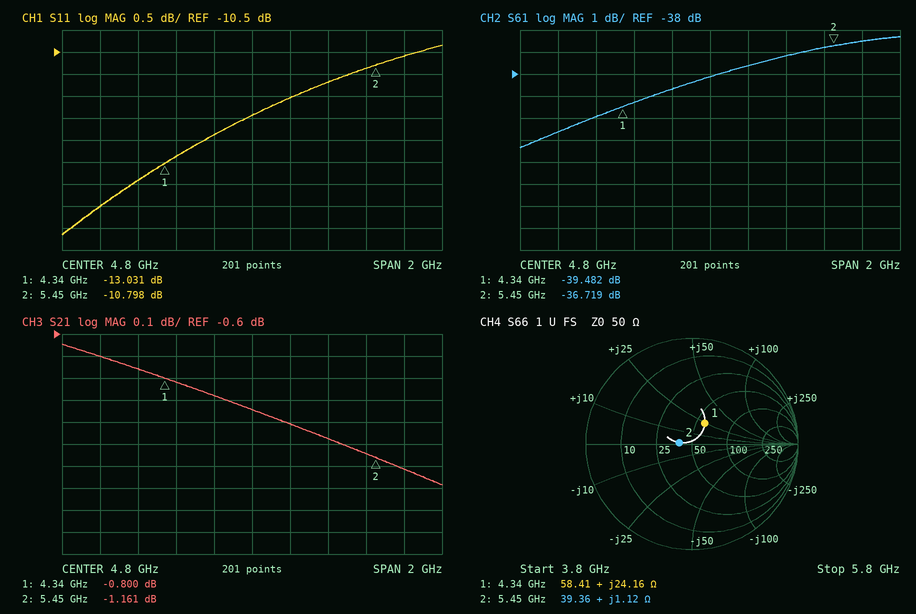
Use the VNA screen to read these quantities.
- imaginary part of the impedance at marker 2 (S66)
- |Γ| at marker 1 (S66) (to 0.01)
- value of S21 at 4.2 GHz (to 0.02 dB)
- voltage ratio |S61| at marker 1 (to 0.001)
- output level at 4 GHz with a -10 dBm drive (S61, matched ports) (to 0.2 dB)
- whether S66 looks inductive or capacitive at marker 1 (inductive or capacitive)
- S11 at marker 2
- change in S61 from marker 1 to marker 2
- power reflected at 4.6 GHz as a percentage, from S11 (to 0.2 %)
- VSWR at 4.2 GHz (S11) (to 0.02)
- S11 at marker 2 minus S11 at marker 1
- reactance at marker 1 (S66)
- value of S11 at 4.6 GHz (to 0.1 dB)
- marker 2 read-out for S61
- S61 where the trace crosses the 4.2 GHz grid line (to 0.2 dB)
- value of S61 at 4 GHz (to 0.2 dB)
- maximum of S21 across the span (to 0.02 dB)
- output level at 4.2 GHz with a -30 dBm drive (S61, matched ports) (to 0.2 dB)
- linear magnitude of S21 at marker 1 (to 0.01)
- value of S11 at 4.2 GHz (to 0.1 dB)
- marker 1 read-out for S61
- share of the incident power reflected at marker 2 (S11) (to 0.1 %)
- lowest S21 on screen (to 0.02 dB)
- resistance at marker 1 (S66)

+1.12 Ω
0.23
-0.76 dB
0.011
-50.6 dBm
inductive
-10.798 dB
2.763 dB
5.8 %
1.54
2.233 dB
+24.16 Ω
-12.4 dB
-36.719 dB
-40.0 dB
-40.6 dB
-0.64 dB
-70.0 dBm
0.91
-13.4 dB
-39.482 dB
8.3 %
-1.28 dB
58.41 Ω
